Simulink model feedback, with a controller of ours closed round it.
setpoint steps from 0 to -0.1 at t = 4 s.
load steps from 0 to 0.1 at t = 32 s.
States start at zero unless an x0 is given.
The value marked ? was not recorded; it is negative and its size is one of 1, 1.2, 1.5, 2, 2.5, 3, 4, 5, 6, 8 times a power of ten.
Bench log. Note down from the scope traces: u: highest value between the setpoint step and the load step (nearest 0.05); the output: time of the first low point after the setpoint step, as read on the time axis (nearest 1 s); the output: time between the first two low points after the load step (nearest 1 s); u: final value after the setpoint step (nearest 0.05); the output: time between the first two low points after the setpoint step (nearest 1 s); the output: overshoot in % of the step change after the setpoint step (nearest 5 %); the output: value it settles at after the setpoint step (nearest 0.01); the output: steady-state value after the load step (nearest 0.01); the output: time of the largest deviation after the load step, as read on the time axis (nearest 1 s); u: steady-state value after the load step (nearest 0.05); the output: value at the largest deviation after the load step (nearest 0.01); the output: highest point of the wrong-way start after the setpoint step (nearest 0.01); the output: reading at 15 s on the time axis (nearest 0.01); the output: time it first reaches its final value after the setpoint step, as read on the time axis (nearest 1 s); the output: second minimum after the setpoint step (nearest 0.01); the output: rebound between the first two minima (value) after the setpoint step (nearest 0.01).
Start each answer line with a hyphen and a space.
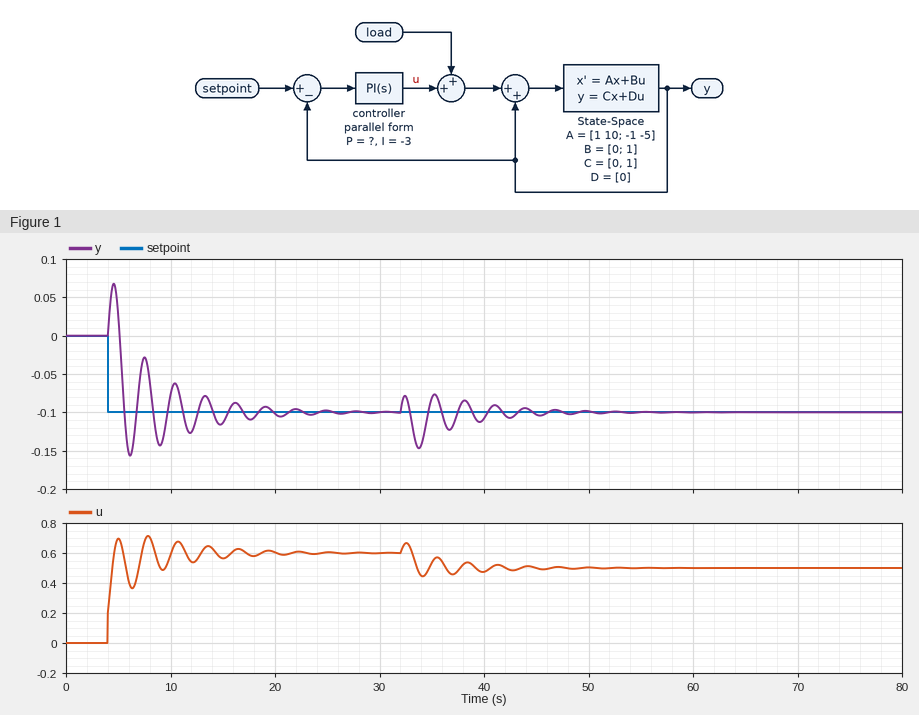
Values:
- 0.70
- 6 s
- 3 s
- 0.60
- 3 s
- 55 %
- -0.10
- -0.10
- 34 s
- 0.50
- -0.15
- 0.07
- -0.11
- 6 s
- -0.14
- -0.03
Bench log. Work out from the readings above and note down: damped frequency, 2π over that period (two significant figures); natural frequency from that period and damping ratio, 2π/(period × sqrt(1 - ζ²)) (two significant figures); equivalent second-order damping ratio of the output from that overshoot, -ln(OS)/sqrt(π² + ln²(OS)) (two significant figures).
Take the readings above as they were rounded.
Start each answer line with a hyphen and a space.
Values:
- 2.1 rad/s
- 2.1 rad/s
- 0.19
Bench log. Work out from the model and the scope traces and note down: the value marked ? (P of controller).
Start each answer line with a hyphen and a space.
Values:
- -2
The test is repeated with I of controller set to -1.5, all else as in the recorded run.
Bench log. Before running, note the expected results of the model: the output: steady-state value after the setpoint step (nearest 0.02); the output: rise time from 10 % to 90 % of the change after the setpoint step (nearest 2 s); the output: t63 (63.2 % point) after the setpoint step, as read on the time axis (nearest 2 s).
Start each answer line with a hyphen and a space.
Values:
- -0.10
- 8 s
- 6 s
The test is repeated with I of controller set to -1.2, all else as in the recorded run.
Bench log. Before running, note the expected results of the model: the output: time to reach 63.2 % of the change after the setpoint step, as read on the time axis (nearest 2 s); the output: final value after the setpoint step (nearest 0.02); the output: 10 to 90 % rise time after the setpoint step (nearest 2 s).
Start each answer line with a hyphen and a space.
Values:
- 6 s
- -0.10
- 10 s
